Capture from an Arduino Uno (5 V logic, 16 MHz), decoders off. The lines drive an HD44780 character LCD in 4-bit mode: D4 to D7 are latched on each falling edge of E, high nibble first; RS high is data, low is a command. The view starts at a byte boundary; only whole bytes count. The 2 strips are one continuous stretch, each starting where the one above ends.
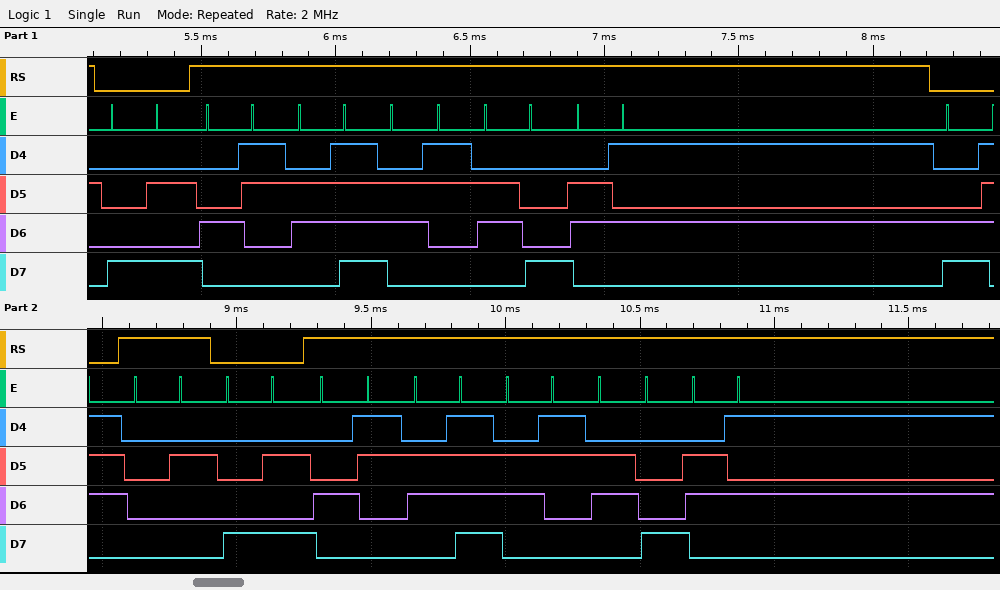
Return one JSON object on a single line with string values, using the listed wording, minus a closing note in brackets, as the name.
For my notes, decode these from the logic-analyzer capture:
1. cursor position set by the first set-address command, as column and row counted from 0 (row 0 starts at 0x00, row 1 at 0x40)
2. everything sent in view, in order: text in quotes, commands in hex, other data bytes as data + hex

{"cursor position set by the first set-address command, as column and row counted from 0": "column 10, row 0", "everything sent in view, in order: text in quotes, commands in hex, other data bytes as data + hex": "0x8A \"Coche\" 0xC7 data 02 0x8A \"Coche\""}
